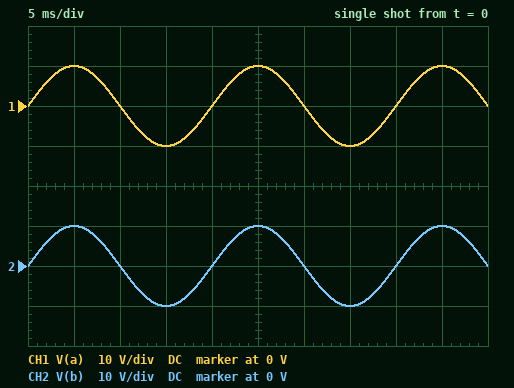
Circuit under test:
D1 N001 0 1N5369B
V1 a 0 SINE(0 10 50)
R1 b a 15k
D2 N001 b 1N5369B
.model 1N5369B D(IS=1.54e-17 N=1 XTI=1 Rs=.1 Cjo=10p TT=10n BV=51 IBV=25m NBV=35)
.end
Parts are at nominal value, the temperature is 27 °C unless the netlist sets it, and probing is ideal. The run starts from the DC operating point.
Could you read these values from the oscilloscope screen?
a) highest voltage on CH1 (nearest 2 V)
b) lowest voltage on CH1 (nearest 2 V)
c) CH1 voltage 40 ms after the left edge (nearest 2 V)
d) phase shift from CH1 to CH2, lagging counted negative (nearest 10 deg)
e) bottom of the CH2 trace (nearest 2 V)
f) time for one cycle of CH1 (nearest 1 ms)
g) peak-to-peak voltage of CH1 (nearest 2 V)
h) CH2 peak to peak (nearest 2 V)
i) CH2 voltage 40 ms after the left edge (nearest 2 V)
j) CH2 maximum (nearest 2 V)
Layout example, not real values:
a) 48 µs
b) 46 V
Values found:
a) 10 V
b) -10 V
c) 0 V
d) 0 deg
e) -10 V
f) 20 ms
g) 20 V
h) 20 V
i) 0 V
j) 10 V
